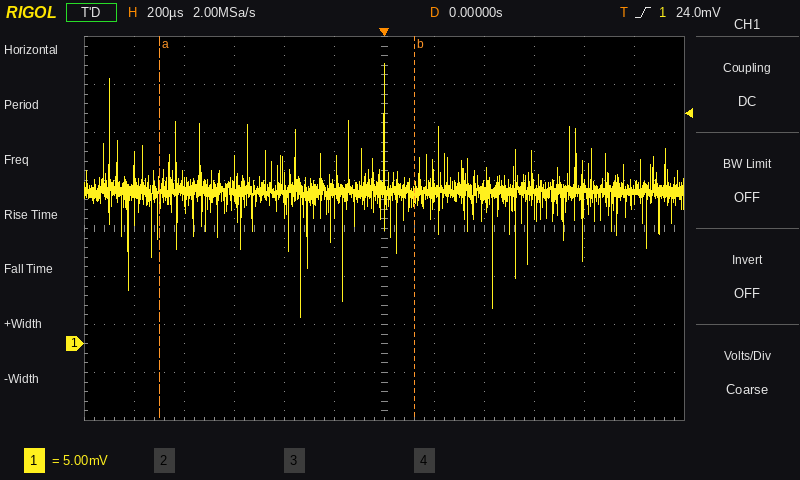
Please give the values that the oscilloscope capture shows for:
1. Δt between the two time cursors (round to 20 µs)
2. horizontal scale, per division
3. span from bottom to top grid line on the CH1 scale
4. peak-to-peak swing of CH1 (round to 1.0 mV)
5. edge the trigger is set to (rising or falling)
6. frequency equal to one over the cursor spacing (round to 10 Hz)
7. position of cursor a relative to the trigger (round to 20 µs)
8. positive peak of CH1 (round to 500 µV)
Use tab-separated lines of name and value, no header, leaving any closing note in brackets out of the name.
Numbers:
Δt between the two time cursors	1.02 ms
horizontal scale, per division	200 µs
span from bottom to top grid line on the CH1 scale	40 mV
peak-to-peak swing of CH1	26.0 mV
edge the trigger is set to	rising
frequency equal to one over the cursor spacing	980 Hz
position of cursor a relative to the trigger	-900 µs
positive peak of CH1	29.0 mV
